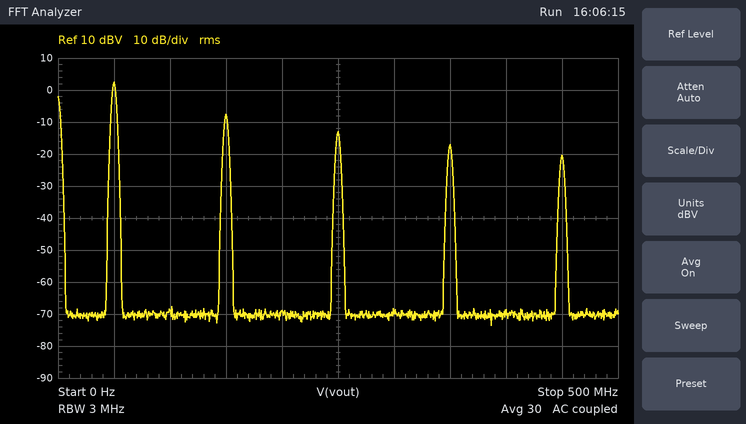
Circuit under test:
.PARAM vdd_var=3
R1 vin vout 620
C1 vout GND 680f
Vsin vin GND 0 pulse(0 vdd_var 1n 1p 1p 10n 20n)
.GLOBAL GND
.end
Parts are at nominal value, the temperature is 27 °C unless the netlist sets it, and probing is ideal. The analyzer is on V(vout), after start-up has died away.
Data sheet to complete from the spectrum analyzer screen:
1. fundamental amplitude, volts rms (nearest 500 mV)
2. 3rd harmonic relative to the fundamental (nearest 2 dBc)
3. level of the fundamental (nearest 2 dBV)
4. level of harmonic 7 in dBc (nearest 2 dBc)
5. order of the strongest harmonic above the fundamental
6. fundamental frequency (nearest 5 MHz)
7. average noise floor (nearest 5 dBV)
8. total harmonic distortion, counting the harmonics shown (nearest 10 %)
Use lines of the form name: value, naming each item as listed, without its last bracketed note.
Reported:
fundamental amplitude, volts rms: 1.5 V
3rd harmonic relative to the fundamental: -10 dBc
level of the fundamental: 2 dBV
level of harmonic 7 in dBc: -20 dBc
order of the strongest harmonic above the fundamental: 3
fundamental frequency: 50 MHz
average noise floor: -70 dBV
total harmonic distortion, counting the harmonics shown: 40 %
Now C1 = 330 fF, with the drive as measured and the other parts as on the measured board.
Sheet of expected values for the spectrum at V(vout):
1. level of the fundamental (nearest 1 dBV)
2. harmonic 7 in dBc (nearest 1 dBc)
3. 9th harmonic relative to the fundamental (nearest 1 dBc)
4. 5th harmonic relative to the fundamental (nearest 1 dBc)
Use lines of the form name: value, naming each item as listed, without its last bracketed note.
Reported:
level of the fundamental: 3 dBV
harmonic 7 in dBc: -18 dBc
9th harmonic relative to the fundamental: -20 dBc
5th harmonic relative to the fundamental: -14 dBc
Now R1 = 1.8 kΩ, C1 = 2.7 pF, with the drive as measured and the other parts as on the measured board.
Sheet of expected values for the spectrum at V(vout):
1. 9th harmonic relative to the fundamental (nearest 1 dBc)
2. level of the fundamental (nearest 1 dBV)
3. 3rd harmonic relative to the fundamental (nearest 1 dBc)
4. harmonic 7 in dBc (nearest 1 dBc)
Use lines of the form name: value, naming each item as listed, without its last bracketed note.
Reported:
9th harmonic relative to the fundamental: -37 dBc
level of the fundamental: -3 dBV
3rd harmonic relative to the fundamental: -18 dBc
harmonic 7 in dBc: -32 dBc
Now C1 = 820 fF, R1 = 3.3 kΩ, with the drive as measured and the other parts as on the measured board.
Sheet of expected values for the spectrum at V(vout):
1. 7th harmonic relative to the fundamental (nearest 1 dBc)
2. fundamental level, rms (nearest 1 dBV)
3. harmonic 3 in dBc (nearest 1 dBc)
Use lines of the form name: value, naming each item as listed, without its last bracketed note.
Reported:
7th harmonic relative to the fundamental: -30 dBc
fundamental level, rms: 0 dBV
harmonic 3 in dBc: -16 dBc
